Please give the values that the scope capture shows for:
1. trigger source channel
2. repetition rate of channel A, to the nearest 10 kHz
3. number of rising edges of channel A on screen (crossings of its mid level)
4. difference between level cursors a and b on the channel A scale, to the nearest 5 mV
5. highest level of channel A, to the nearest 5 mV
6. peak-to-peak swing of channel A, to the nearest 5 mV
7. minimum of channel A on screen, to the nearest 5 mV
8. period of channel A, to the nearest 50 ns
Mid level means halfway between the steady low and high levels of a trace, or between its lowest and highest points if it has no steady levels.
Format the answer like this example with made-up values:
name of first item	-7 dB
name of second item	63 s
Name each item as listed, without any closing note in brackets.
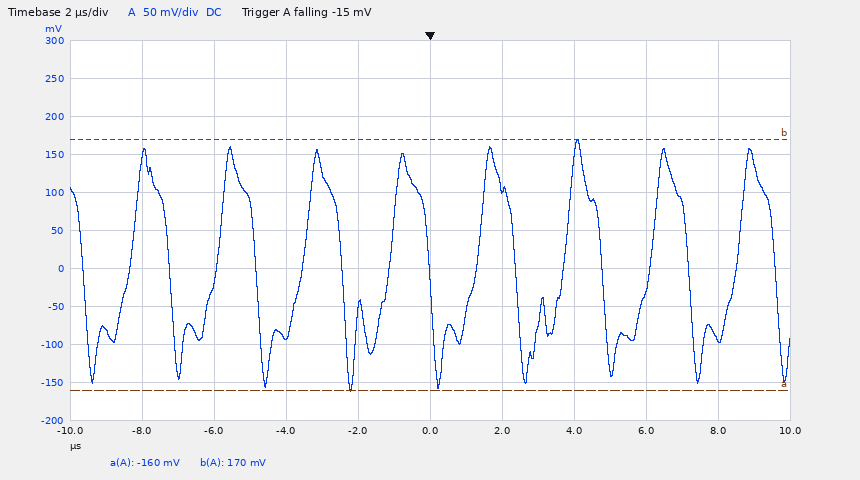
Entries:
trigger source channel	channel A
repetition rate of channel A, to the nearest 10 kHz	420 kHz
number of rising edges of channel A on screen	8
difference between level cursors a and b on the channel A scale, to the nearest 5 mV	330 mV
highest level of channel A, to the nearest 5 mV	170 mV
peak-to-peak swing of channel A, to the nearest 5 mV	330 mV
minimum of channel A on screen, to the nearest 5 mV	-160 mV
period of channel A, to the nearest 50 ns	2.40 µs
